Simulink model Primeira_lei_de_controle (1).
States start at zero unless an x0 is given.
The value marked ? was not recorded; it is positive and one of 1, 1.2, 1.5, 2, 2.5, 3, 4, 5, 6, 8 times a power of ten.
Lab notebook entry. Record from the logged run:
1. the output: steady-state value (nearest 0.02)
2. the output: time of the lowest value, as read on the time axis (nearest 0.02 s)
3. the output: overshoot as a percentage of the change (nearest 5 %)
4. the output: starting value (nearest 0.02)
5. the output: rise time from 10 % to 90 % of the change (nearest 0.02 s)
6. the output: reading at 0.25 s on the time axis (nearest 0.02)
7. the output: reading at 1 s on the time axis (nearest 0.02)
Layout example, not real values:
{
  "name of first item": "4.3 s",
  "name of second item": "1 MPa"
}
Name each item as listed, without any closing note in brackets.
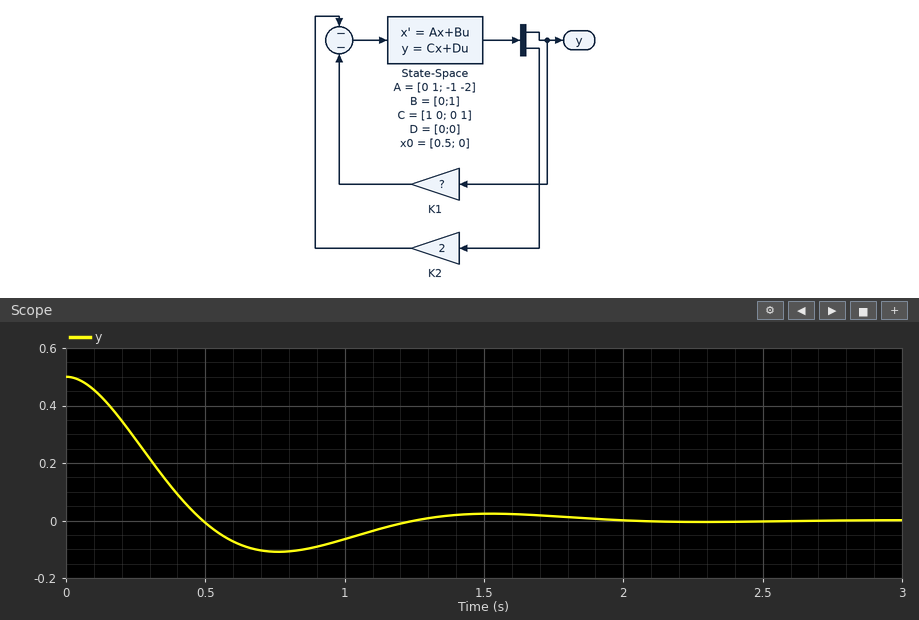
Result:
{
  "the output: steady-state value": "0.00",
  "the output: time of the lowest value, as read on the time axis": "0.76 s",
  "the output: overshoot as a percentage of the change": "20 %",
  "the output: starting value": "0.50",
  "the output: rise time from 10 % to 90 % of the change": "0.34 s",
  "the output: reading at 0.25 s on the time axis": "0.28",
  "the output: reading at 1 s on the time axis": "-0.06"
}
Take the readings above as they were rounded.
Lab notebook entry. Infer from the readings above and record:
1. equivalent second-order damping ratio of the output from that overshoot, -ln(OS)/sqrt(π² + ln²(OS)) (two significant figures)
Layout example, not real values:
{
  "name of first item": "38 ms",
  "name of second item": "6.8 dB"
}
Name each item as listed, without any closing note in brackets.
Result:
{
  "equivalent second-order damping ratio of the output from that overshoot, -ln(OS)/sqrt(π² + ln²(OS))": "0.46"
}
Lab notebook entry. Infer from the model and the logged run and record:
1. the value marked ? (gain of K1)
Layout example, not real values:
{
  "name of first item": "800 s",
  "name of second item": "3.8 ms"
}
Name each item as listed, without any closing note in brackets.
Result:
{
  "the value marked ?": "20"
}
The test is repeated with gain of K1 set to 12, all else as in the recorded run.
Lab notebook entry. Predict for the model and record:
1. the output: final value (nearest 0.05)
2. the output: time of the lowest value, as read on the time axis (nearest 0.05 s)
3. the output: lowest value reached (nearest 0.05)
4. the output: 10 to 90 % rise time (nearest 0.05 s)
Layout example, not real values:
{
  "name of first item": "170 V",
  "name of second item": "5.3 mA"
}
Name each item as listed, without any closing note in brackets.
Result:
{
  "the output: final value": "0.00",
  "the output: time of the lowest value, as read on the time axis": "1.05 s",
  "the output: lowest value reached": "-0.05",
  "the output: 10 to 90 % rise time": "0.50 s"
}
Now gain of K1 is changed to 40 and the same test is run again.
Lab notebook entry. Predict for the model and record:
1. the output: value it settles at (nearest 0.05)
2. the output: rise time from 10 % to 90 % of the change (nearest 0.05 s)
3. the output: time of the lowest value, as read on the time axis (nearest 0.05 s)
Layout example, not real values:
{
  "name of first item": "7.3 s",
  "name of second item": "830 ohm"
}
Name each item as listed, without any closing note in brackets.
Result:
{
  "the output: value it settles at": "0.00",
  "the output: rise time from 10 % to 90 % of the change": "0.20 s",
  "the output: time of the lowest value, as read on the time axis": "0.50 s"
}
